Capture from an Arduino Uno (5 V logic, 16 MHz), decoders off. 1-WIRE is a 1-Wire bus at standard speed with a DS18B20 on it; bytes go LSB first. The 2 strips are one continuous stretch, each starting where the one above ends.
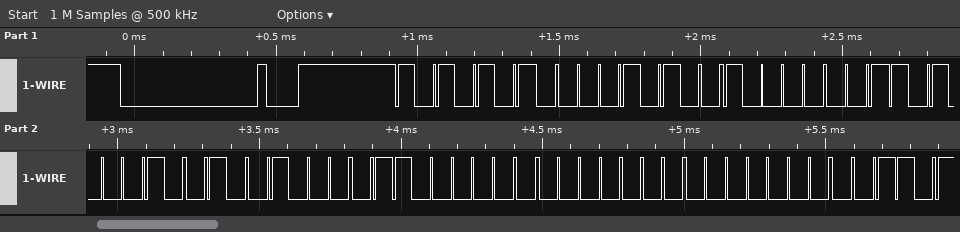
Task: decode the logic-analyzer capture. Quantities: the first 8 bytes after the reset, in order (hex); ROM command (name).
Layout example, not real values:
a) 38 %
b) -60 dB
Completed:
a) 55 28 81 45 12 06 00 00
b) Match ROM
